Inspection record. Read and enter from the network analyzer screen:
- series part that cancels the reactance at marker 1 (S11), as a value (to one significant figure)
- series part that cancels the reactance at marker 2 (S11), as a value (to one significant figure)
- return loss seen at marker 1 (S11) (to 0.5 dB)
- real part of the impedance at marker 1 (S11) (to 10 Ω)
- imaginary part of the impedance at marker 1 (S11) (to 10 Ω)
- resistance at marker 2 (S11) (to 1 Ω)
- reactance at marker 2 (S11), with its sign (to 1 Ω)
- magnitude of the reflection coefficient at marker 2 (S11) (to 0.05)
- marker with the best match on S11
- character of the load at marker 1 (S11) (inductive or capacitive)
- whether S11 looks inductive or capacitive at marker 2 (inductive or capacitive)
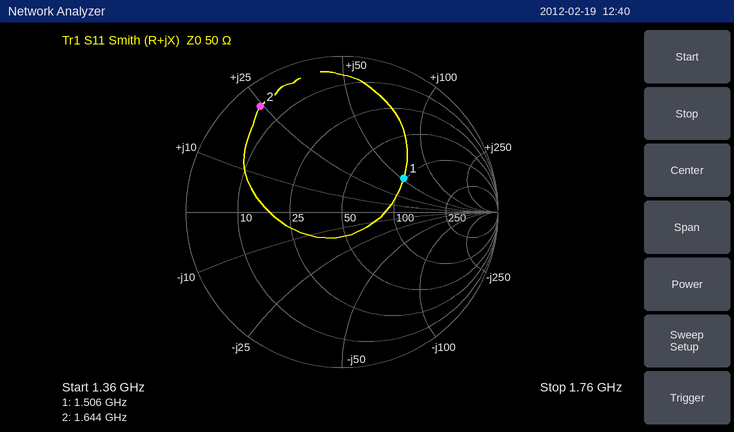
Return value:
2 pF
4 pF
7.0 dB
100 Ω
+50 Ω
5 Ω
+24 Ω
0.85
marker 1
inductive
inductive
